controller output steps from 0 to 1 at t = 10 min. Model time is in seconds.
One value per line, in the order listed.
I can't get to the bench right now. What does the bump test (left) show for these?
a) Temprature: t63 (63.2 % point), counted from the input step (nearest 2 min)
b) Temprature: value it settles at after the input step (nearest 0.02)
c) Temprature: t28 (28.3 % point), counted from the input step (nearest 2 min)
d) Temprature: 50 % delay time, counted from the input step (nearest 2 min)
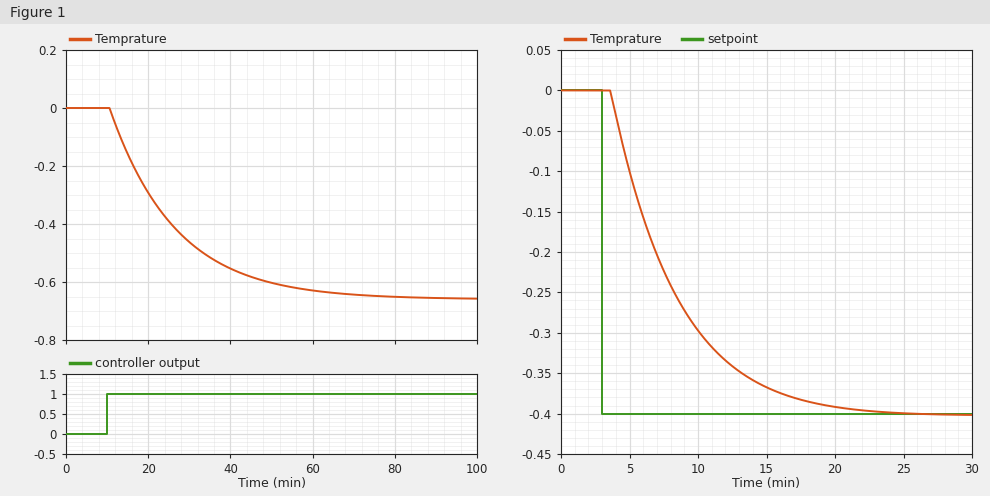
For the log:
16 min
-0.66
6 min
12 min
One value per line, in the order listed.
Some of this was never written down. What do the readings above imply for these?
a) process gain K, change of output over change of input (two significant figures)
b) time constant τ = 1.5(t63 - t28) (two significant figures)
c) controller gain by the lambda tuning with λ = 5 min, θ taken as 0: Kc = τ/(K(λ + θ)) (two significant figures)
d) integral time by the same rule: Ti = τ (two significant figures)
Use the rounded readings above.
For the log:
-0.66
15 min
-4.5
15 min
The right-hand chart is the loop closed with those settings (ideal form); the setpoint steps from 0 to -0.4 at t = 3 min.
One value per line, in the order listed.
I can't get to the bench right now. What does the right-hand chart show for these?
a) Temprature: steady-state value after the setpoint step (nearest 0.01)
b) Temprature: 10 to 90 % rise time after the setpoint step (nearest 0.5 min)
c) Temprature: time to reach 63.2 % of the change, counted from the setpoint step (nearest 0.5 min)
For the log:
-0.40
10.0 min
5.5 min
